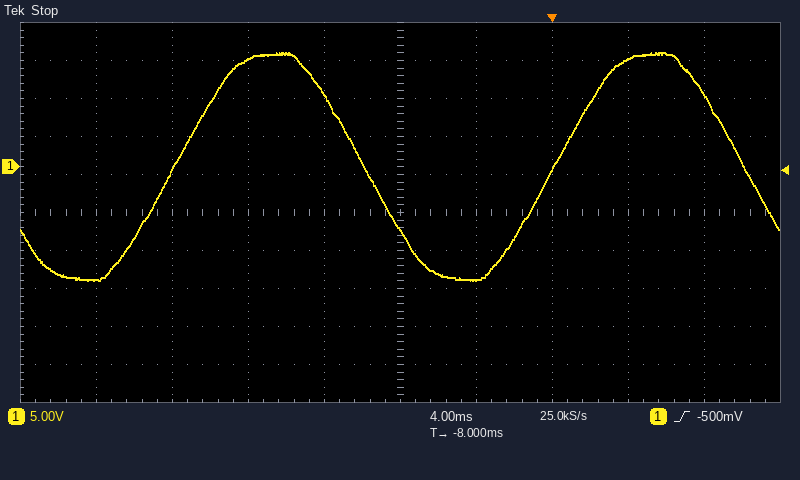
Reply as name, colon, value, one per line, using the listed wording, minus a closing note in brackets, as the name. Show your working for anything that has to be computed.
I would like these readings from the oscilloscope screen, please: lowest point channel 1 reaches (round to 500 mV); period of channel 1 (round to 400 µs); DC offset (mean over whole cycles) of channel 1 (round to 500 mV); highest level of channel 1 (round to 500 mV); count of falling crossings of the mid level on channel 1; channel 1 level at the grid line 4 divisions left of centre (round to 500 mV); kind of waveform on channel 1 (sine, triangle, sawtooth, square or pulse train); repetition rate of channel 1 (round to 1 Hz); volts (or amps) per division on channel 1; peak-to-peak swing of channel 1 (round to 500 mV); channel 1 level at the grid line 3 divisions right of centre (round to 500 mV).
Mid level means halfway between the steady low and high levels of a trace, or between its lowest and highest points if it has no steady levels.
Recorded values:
lowest point channel 1 reaches: -15.0 V
period of channel 1: 20.0 ms
DC offset (mean over whole cycles) of channel 1: (15.0 V + (-15.0 V)) / 2 ≈ 0.0 V
highest level of channel 1: 15.0 V
count of falling crossings of the mid level on channel 1: 2
channel 1 level at the grid line 4 divisions left of centre: -15.0 V
kind of waveform on channel 1: sine
repetition rate of channel 1: 1 / 20.0 ms ≈ 50 Hz
volts (or amps) per division on channel 1: 5 V
peak-to-peak swing of channel 1: 15.0 V − (-15.0 V) = 30.0 V
channel 1 level at the grid line 3 divisions right of centre: 14.0 V
